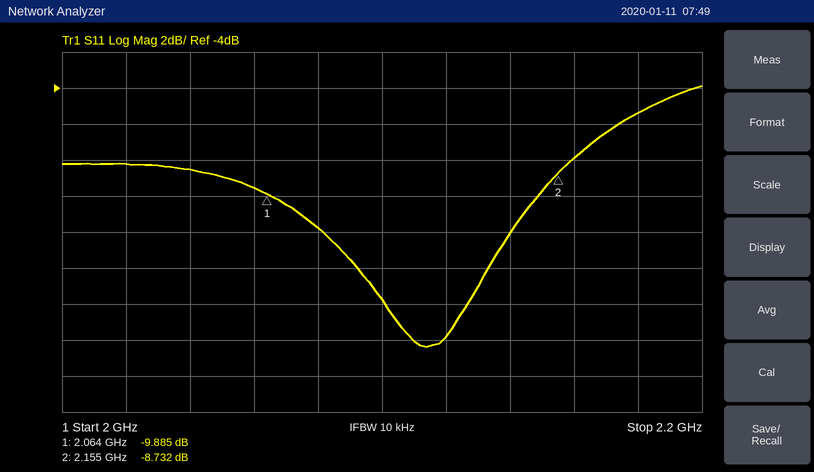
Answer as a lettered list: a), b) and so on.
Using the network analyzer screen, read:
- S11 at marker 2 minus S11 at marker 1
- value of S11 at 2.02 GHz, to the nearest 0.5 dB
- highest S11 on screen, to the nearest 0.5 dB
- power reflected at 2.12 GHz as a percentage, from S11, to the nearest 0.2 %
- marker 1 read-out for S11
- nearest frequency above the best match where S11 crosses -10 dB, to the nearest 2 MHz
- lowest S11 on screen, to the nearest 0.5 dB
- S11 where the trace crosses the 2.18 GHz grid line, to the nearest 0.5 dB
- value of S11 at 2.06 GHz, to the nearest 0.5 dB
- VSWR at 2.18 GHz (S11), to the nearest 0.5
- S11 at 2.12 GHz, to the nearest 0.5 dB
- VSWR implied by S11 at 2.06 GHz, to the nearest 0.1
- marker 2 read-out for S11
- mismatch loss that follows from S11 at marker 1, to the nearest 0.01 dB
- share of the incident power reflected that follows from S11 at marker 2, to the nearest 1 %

a) 1.153 dB
b) -8.0 dB
c) -4.0 dB
d) 1.6 %
e) -9.885 dB
f) 2.148 GHz
g) -18.5 dB
h) -5.5 dB
i) -9.5 dB
j) 3.5
k) -18.0 dB
l) 2.0
m) -8.732 dB
n) 0.47 dB
o) 13 %
